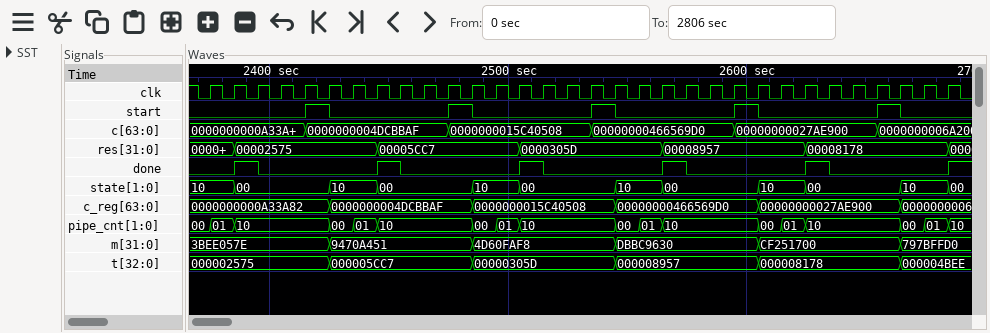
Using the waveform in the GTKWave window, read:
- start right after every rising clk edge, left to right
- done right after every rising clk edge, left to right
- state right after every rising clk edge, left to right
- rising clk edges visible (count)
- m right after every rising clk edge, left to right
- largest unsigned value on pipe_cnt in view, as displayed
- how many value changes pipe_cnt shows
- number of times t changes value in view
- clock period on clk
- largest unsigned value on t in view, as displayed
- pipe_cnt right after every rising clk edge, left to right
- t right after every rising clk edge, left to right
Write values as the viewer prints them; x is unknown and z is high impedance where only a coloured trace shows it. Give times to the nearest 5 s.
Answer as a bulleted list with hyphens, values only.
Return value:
- 0 0 0 0 1 0 0 0 0 0 1 0 0 0 0 0 1 0 0 0 0 0 1 0 0 0 0 0 1 0 0 0
- 0 1 0 0 0 0 0 1 0 0 0 0 0 1 0 0 0 0 0 1 0 0 0 0 0 1 0 0 0 0 0 1
- 10, 00, 00, 00, 00, 10, 10, 00, 00, 00, 00, 10, 10, 00, 00, 00, 00, 10, 10, 00, 00, 00, 00, 10, 10, 00, 00, 00, 00, 10, 10, 00
- 32
- 3BEE057E, 3BEE057E, 3BEE057E, 3BEE057E, 3BEE057E, 9470A451, 9470A451, 9470A451, 9470A451, 9470A451, 9470A451, 4D60FAF8, 4D60FAF8, 4D60FAF8, 4D60FAF8, 4D60FAF8, 4D60FAF8, DBBC9630, DBBC9630, DBBC9630, DBBC9630, DBBC9630, DBBC9630, CF251700, CF251700, CF251700, CF251700, CF251700, CF251700, 797BFFD0, 797BFFD0, 797BFFD0
- 10
- 17
- 5
- 10 s
- 000008957
- 01, 10, 10, 10, 10, 00, 01, 10, 10, 10, 10, 00, 01, 10, 10, 10, 10, 00, 01, 10, 10, 10, 10, 00, 01, 10, 10, 10, 10, 00, 01, 10
- 000002575, 000002575, 000002575, 000002575, 000002575, 000005CC7, 000005CC7, 000005CC7, 000005CC7, 000005CC7, 000005CC7, 00000305D, 00000305D, 00000305D, 00000305D, 00000305D, 00000305D, 000008957, 000008957, 000008957, 000008957, 000008957, 000008957, 000008178, 000008178, 000008178, 000008178, 000008178, 000008178, 000004BEE, 000004BEE, 000004BEE
